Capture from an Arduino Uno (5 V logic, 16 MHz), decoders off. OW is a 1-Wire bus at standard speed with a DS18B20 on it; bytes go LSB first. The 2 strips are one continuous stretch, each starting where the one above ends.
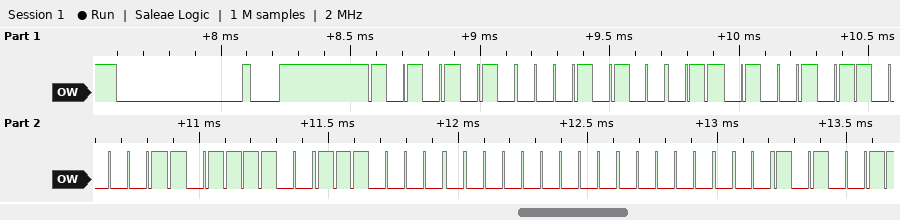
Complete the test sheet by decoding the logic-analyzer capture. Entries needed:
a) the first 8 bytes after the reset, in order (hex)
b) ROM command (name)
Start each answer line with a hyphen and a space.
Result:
- 55 28 96 86 3D 07 00 00
- Match ROM
